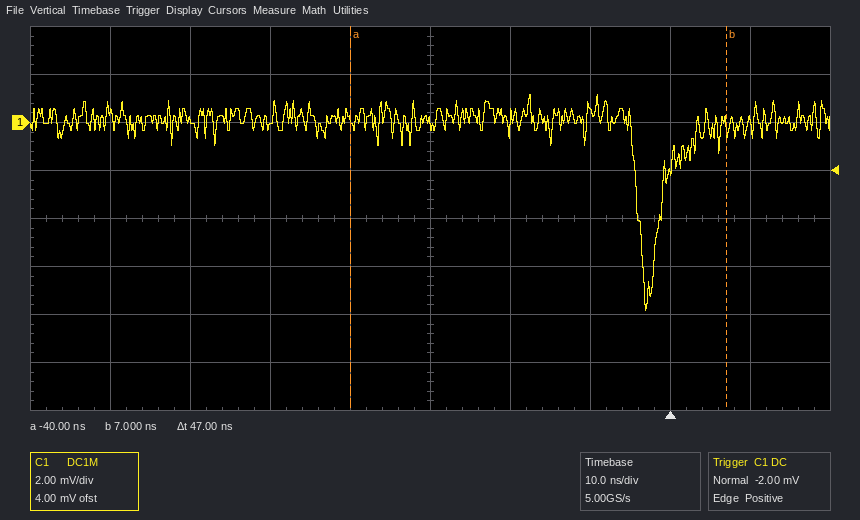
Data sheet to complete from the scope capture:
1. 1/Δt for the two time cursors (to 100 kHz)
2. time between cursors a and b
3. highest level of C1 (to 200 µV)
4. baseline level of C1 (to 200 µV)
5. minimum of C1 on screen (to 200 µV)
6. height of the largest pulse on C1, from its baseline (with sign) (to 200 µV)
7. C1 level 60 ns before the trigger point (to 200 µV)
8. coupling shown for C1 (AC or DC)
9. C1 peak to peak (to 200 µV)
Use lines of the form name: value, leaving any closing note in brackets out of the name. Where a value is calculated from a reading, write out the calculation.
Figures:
1/Δt for the two time cursors: 1 / 47 ns ≈ 21.3 MHz
time between cursors a and b: 47 ns
highest level of C1: 1.2 mV
baseline level of C1: 200 µV
minimum of C1 on screen: -7.8 mV
height of the largest pulse on C1, from its baseline (with sign): -7.8 mV − (200 µV) = -8.0 mV
C1 level 60 ns before the trigger point: 200 µV
coupling shown for C1: DC
C1 peak to peak: 1.2 mV − (-7.8 mV) = 9.0 mV
